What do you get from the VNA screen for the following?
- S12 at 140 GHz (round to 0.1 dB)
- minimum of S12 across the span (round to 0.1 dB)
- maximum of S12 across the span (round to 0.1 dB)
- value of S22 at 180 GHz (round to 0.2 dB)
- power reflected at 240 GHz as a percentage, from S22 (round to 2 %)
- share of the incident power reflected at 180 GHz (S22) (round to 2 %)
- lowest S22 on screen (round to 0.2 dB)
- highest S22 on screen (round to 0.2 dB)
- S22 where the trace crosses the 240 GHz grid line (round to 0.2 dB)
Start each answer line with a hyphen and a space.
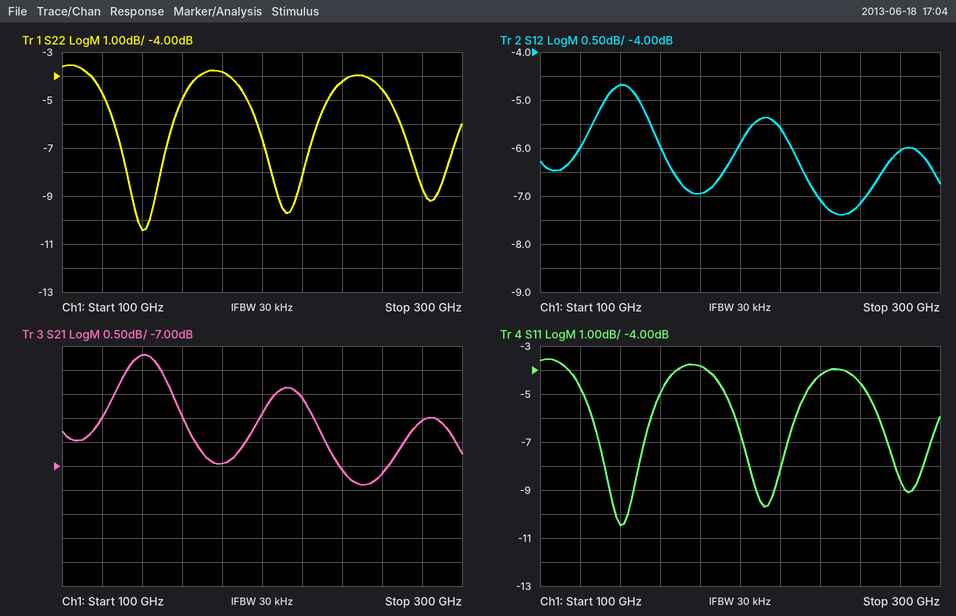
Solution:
- -4.7 dB
- -7.4 dB
- -4.7 dB
- -3.8 dB
- 38 %
- 42 %
- -10.4 dB
- -3.6 dB
- -4.2 dB
